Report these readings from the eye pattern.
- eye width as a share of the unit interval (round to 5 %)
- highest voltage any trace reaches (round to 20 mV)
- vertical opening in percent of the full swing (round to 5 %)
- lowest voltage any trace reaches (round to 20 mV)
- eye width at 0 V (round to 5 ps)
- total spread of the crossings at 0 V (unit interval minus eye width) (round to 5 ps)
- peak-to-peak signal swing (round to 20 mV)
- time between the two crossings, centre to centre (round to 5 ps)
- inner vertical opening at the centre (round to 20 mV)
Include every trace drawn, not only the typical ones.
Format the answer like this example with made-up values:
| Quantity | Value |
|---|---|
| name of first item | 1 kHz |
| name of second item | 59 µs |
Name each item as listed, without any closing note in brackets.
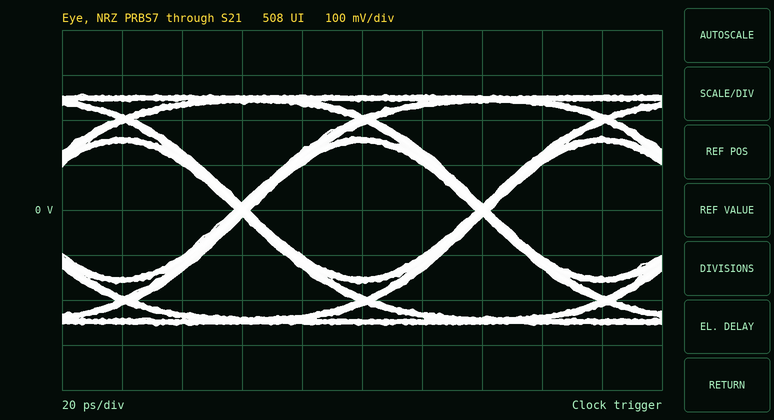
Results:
| Quantity | Value |
|---|---|
| eye width as a share of the unit interval | 95 % |
| highest voltage any trace reaches | 260 mV |
| vertical opening in percent of the full swing | 60 % |
| lowest voltage any trace reaches | -260 mV |
| eye width at 0 V | 75 ps |
| total spread of the crossings at 0 V (unit interval minus eye width) | 5 ps |
| peak-to-peak signal swing | 520 mV |
| time between the two crossings, centre to centre | 80 ps |
| inner vertical opening at the centre | 300 mV |
